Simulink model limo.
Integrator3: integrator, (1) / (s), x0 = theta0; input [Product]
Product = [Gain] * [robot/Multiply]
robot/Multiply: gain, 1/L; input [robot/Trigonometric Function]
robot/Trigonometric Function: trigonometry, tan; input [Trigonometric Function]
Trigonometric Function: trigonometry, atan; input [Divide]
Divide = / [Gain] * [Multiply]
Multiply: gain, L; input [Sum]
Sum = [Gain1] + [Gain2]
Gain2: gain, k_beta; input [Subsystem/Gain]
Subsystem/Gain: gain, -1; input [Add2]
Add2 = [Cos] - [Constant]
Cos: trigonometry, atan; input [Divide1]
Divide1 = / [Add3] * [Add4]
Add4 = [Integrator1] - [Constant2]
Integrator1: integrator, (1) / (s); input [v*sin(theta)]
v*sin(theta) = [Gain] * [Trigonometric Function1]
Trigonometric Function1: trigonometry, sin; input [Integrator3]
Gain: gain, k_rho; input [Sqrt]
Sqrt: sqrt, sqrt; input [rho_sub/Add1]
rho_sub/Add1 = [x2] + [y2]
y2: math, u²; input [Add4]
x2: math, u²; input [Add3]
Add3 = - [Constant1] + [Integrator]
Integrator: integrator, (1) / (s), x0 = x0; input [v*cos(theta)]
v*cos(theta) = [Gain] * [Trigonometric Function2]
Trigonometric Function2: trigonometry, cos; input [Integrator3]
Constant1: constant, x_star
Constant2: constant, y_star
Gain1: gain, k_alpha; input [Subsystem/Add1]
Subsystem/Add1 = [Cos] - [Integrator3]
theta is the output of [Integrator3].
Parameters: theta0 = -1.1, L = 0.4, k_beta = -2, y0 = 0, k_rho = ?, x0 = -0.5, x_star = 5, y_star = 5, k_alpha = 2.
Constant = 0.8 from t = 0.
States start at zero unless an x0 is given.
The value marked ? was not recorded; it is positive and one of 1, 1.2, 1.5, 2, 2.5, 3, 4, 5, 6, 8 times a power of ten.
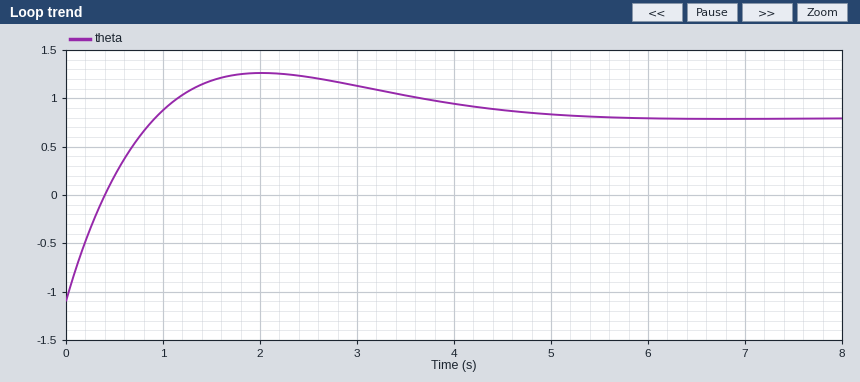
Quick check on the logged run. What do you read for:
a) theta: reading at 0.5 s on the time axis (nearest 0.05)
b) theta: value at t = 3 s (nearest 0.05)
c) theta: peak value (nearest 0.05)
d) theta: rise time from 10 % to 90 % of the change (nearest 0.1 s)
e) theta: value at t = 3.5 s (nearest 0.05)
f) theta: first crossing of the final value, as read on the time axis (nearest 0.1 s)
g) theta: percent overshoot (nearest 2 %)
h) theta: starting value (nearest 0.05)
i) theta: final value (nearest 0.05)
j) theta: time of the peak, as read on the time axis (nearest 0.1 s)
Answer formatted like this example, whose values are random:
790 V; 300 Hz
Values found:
0.20; 1.15; 1.25; 0.7 s; 1.05; 0.9 s; 24 %; -1.10; 0.80; 2.0 s
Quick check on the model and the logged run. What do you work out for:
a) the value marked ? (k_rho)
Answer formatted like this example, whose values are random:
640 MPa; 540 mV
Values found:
0.5
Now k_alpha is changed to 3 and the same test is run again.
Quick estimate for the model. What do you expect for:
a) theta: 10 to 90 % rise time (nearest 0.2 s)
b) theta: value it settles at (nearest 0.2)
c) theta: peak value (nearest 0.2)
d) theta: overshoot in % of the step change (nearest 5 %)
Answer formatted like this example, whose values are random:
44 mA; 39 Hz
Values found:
0.6 s; 0.8; 1.0; 15 %
